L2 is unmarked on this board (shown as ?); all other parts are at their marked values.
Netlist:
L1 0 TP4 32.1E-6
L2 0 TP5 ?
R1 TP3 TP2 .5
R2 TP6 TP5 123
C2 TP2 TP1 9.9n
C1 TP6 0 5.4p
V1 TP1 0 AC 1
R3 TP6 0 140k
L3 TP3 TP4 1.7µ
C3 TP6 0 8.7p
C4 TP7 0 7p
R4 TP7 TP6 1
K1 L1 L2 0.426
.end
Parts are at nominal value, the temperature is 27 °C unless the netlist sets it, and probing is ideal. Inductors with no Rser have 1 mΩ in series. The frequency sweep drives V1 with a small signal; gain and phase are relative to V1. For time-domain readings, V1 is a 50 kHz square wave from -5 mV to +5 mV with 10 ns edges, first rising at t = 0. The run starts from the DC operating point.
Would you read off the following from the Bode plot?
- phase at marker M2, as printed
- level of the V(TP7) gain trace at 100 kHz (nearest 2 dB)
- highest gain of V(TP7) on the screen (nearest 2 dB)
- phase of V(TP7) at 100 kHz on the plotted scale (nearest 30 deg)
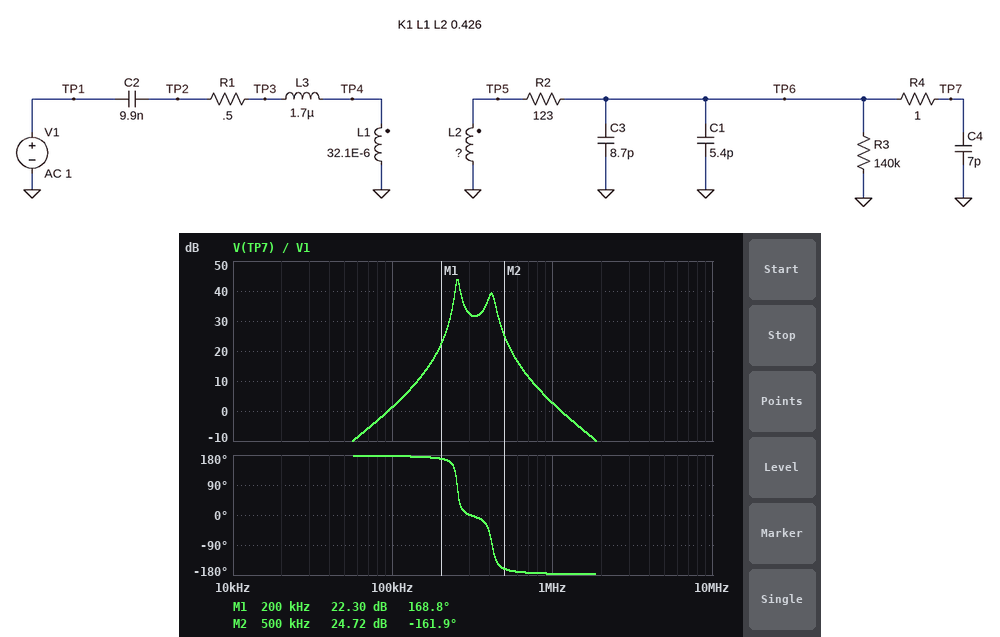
-161.9 deg
2 dB
44 dB
180 deg
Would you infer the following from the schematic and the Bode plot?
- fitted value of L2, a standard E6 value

10 mH
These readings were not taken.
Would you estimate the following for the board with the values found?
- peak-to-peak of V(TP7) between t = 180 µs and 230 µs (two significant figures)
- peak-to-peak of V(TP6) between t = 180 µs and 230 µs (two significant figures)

490 mV
490 mV
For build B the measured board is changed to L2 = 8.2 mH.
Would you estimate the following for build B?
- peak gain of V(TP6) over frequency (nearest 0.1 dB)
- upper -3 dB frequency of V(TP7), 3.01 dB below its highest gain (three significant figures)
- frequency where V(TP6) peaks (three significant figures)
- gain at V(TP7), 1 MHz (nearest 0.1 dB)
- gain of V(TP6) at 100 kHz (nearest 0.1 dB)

45.3 dB
264 kHz
258 kHz
3.7 dB
0.5 dB
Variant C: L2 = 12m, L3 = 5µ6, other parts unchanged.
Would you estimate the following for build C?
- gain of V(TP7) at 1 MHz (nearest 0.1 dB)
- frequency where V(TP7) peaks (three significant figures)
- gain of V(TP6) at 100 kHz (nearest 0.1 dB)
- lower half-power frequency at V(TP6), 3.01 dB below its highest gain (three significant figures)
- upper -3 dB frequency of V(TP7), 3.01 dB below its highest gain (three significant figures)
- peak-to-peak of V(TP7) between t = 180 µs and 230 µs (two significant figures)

0.2 dB
239 kHz
2.6 dB
232 kHz
249 kHz
390 mV
